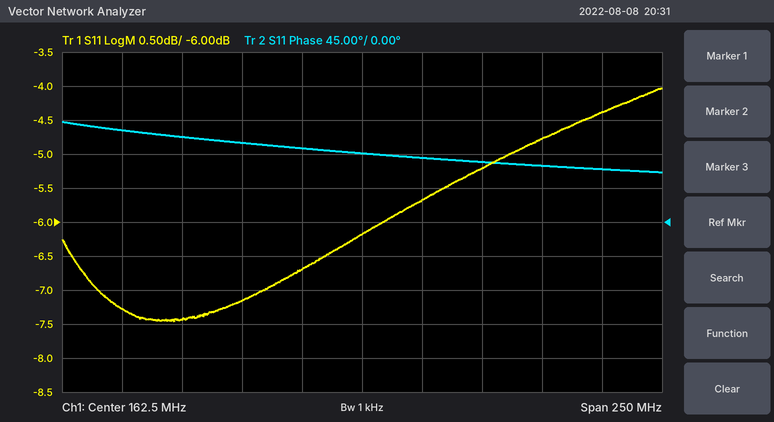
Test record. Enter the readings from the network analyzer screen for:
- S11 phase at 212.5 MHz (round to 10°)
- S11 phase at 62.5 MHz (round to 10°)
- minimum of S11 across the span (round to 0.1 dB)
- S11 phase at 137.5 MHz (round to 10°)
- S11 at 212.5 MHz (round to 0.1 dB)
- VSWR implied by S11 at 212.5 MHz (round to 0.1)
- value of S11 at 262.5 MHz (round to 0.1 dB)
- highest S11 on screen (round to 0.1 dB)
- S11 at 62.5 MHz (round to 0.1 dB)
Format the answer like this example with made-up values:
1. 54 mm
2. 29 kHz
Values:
1. 80°
2. 120°
3. -7.5 dB
4. 100°
5. -5.2 dB
6. 3.4
7. -4.4 dB
8. -4.0 dB
9. -7.3 dB
